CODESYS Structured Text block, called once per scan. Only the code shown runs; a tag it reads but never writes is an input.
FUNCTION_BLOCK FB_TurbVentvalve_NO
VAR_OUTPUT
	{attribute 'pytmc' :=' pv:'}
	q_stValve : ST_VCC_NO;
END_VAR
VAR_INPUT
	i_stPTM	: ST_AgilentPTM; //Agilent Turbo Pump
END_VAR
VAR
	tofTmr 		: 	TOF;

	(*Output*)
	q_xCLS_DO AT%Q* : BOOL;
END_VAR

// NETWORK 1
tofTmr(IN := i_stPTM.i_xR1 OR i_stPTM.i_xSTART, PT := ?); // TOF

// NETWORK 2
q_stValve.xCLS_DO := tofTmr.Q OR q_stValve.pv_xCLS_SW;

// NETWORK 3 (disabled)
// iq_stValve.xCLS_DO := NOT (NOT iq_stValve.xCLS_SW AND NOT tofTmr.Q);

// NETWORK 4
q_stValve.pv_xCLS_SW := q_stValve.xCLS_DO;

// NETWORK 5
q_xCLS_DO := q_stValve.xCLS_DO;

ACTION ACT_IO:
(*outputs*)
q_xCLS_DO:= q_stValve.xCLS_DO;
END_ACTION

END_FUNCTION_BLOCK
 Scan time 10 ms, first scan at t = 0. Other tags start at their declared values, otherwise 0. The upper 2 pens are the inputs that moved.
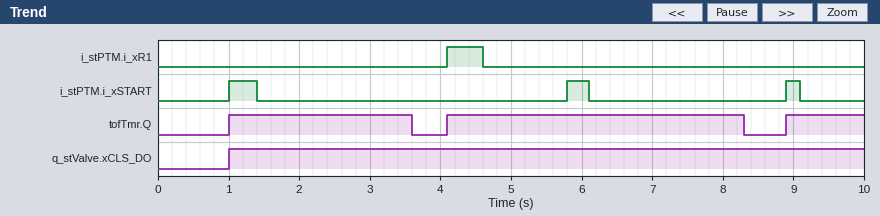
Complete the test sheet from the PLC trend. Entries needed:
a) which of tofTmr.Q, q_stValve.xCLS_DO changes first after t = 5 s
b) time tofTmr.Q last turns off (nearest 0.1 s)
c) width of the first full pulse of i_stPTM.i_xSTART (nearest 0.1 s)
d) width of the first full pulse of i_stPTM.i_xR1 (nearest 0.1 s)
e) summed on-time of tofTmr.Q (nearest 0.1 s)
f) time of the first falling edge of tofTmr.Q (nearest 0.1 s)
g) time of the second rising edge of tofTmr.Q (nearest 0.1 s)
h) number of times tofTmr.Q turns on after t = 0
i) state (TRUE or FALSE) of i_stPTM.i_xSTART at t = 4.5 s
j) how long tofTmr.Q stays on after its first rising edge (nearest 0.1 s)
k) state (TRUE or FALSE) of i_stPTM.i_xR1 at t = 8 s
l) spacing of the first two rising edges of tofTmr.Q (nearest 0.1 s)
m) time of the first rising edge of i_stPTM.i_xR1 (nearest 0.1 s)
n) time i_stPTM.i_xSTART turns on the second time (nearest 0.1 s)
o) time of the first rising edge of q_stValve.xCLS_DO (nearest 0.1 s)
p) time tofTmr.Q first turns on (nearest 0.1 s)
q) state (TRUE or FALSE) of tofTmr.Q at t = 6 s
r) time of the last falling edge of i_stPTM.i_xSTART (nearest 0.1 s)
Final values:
tofTmr.Q
8.3 s
0.4 s
0.5 s
7.9 s
3.6 s
4.1 s
3
FALSE
2.6 s
FALSE
3.1 s
4.1 s
5.8 s
1.0 s
1.0 s
TRUE
9.1 s
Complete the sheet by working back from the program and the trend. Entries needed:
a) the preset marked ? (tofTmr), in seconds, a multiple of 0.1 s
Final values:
2.2 s
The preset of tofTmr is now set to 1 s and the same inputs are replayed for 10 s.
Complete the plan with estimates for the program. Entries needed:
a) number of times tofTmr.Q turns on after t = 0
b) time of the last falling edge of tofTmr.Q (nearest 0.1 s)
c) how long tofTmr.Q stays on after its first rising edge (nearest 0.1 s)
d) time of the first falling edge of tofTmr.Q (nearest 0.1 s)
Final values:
4
7.1 s
1.4 s
2.4 s
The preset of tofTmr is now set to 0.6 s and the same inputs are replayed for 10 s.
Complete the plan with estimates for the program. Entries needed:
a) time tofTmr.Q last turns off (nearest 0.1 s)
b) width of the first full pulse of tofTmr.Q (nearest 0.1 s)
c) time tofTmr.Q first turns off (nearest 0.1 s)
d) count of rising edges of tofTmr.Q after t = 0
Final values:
9.7 s
1.0 s
2.0 s
4
